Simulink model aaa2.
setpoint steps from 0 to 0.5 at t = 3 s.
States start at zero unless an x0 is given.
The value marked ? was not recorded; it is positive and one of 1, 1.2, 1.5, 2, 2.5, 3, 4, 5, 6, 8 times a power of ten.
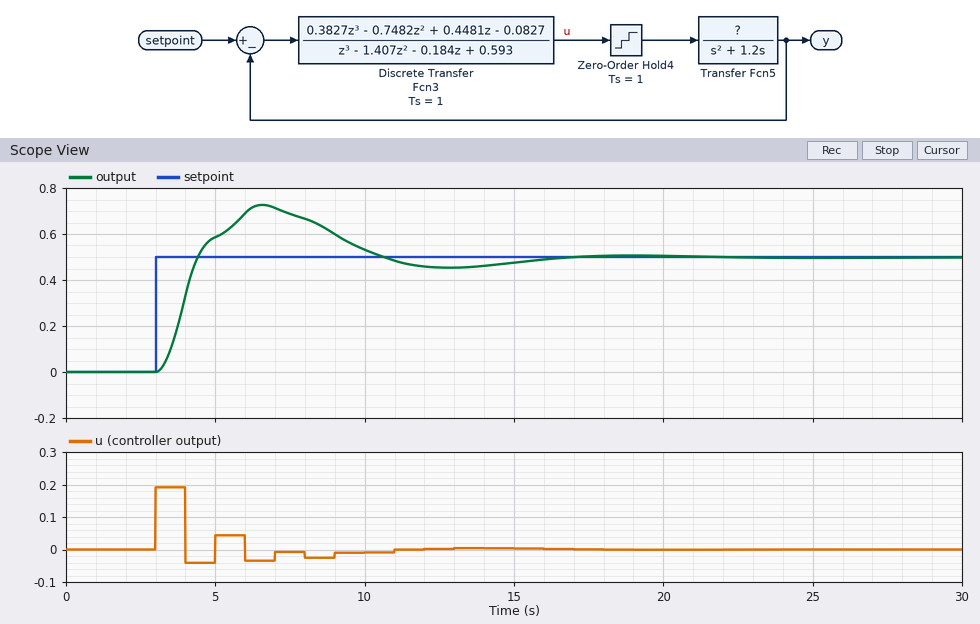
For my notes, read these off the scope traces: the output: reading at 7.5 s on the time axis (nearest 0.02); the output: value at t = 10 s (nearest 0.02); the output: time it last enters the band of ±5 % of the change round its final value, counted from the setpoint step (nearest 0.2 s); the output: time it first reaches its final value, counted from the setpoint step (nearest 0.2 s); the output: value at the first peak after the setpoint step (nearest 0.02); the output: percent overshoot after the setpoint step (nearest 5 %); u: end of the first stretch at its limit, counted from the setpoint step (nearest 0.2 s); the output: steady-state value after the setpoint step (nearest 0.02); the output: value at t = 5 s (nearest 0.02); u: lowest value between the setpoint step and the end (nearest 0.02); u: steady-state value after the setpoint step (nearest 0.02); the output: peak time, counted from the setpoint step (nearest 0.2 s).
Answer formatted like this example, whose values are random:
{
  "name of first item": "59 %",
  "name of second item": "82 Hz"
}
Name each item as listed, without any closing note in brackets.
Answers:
{
  "the output: reading at 7.5 s on the time axis": "0.68",
  "the output: value at t = 10 s": "0.54",
  "the output: time it last enters the band of ±5 % of the change round its final value, counted from the setpoint step": "11.8 s",
  "the output: time it first reaches its final value, counted from the setpoint step": "1.4 s",
  "the output: value at the first peak after the setpoint step": "0.72",
  "the output: percent overshoot after the setpoint step": "45 %",
  "u: end of the first stretch at its limit, counted from the setpoint step": "1.0 s",
  "the output: steady-state value after the setpoint step": "0.50",
  "the output: value at t = 5 s": "0.58",
  "u: lowest value between the setpoint step and the end": "-0.04",
  "u: steady-state value after the setpoint step": "0.00",
  "the output: peak time, counted from the setpoint step": "3.6 s"
}
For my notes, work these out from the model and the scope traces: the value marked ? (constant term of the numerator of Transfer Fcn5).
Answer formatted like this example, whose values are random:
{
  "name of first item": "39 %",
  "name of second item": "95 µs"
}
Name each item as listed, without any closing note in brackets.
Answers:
{
  "the value marked ?": "5"
}
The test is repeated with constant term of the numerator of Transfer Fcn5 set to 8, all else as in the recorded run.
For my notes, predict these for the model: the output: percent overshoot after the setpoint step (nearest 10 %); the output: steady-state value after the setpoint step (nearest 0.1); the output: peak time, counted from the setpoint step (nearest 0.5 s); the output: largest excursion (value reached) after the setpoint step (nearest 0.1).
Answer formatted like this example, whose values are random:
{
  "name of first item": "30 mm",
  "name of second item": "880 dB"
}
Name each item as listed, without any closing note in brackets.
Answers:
{
  "the output: percent overshoot after the setpoint step": "60 %",
  "the output: steady-state value after the setpoint step": "0.5",
  "the output: peak time, counted from the setpoint step": "1.5 s",
  "the output: largest excursion (value reached) after the setpoint step": "0.8"
}
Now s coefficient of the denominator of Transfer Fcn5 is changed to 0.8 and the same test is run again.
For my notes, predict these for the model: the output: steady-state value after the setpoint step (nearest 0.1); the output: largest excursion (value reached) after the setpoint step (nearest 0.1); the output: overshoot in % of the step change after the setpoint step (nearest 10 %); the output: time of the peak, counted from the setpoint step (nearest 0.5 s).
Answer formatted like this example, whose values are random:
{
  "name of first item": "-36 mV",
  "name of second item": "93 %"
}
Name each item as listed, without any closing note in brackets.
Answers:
{
  "the output: steady-state value after the setpoint step": "0.5",
  "the output: largest excursion (value reached) after the setpoint step": "0.8",
  "the output: overshoot in % of the step change after the setpoint step": "60 %",
  "the output: time of the peak, counted from the setpoint step": "3.0 s"
}
